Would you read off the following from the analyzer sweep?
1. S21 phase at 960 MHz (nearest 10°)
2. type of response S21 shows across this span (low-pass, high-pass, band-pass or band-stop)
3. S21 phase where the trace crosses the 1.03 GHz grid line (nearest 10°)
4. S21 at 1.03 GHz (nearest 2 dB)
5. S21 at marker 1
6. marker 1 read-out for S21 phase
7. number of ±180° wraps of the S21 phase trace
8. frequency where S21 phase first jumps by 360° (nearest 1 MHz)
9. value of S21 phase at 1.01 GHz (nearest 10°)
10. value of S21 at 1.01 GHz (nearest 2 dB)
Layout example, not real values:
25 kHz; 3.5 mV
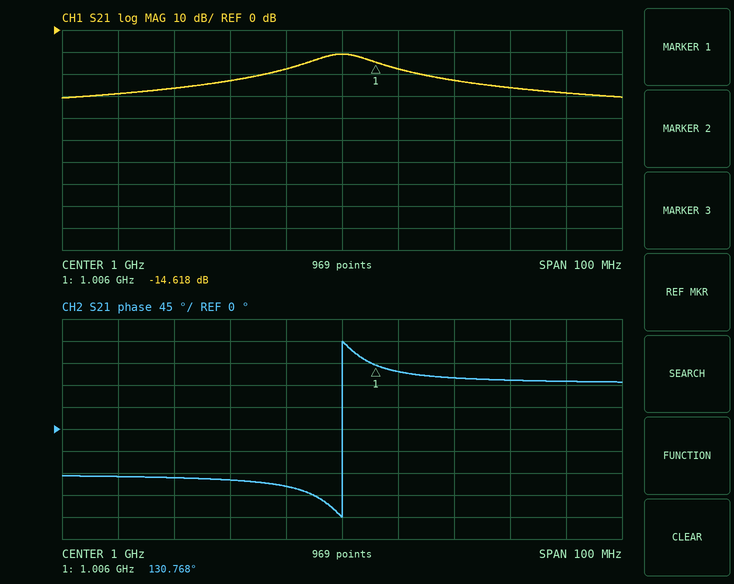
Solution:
-100°; band-pass; 100°; -26 dB; -14.618 dB; 130.768°; 1; 1.000 GHz; 120°; -18 dB
